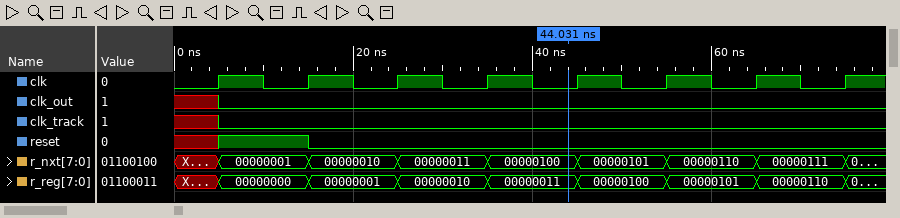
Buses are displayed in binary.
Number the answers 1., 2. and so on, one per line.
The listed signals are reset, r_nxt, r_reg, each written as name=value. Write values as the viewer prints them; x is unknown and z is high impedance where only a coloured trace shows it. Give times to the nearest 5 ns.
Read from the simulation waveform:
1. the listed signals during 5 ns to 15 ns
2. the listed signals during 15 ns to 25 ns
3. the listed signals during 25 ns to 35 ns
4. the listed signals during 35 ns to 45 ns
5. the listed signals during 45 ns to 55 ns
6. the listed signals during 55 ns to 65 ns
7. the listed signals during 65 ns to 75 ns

1. reset=1, r_nxt=00000001, r_reg=00000000
2. reset=0, r_nxt=00000010, r_reg=00000001
3. reset=0, r_nxt=00000011, r_reg=00000010
4. reset=0, r_nxt=00000100, r_reg=00000011
5. reset=0, r_nxt=00000101, r_reg=00000100
6. reset=0, r_nxt=00000110, r_reg=00000101
7. reset=0, r_nxt=00000111, r_reg=00000110
